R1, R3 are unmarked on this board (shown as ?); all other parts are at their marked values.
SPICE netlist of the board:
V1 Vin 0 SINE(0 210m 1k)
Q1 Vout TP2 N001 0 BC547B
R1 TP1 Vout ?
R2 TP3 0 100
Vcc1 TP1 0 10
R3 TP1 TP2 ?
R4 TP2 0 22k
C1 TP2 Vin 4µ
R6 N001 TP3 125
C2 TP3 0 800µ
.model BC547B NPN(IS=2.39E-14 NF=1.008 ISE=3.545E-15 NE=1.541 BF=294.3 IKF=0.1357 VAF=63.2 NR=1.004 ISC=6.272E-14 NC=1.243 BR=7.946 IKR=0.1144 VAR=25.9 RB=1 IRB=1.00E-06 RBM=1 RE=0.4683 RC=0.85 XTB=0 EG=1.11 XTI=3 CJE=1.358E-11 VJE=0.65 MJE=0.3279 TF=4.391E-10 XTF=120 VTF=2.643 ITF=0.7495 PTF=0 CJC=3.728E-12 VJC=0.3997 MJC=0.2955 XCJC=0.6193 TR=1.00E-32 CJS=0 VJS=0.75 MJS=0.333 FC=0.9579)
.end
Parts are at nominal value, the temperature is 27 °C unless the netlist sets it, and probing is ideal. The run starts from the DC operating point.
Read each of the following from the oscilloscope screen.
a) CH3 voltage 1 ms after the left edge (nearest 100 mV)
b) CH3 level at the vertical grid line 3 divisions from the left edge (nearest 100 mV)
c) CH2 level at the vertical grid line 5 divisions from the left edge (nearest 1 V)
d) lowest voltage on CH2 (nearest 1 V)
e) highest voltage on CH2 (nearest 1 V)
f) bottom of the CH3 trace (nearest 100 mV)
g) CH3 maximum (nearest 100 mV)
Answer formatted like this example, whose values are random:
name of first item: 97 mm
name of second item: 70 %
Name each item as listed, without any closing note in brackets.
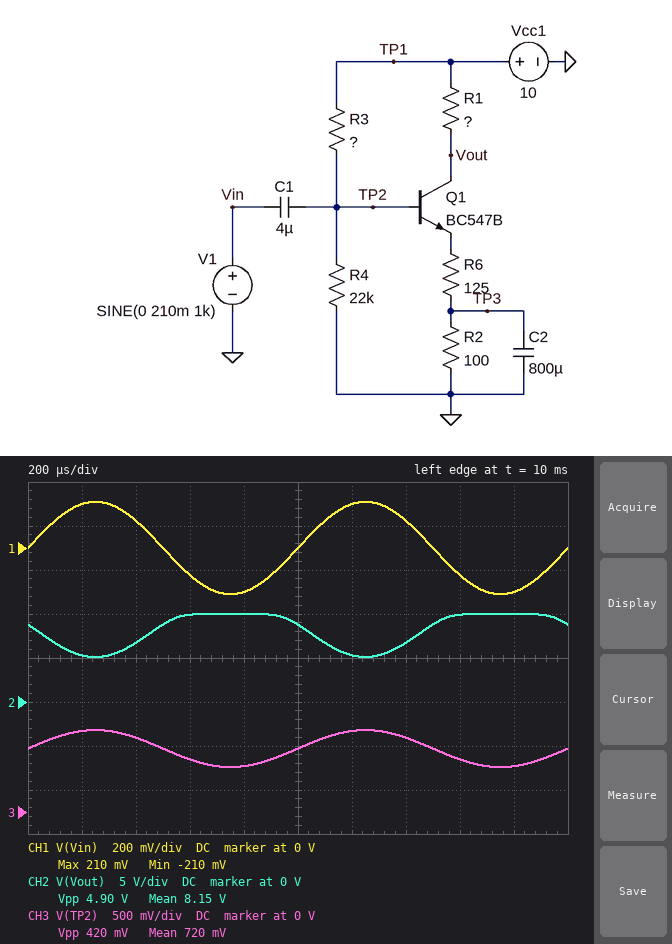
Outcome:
CH3 voltage 1 ms after the left edge: 700 mV
CH3 level at the vertical grid line 3 divisions from the left edge: 600 mV
CH2 level at the vertical grid line 5 divisions from the left edge: 9 V
lowest voltage on CH2: 5 V
highest voltage on CH2: 10 V
bottom of the CH3 trace: 500 mV
CH3 maximum: 900 mV
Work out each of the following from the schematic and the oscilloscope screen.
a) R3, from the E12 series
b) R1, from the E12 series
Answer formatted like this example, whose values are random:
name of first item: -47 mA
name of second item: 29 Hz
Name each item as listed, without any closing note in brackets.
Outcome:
R3, from the E12 series: 270 kΩ
R1, from the E12 series: 2.7 kΩ
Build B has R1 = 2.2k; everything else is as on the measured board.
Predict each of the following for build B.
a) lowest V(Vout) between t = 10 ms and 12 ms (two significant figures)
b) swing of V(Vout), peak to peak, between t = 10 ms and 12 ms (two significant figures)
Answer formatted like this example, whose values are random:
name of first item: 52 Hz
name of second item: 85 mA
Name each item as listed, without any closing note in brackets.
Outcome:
lowest V(Vout) between t = 10 ms and 12 ms: 6.0 V
swing of V(Vout), peak to peak, between t = 10 ms and 12 ms: 4.0 V
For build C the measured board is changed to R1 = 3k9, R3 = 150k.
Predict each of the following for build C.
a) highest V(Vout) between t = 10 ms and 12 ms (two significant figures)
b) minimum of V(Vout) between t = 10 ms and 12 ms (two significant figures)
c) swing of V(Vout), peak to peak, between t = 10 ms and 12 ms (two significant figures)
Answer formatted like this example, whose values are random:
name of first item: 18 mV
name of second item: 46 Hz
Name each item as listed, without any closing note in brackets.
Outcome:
highest V(Vout) between t = 10 ms and 12 ms: 9.7 V
minimum of V(Vout) between t = 10 ms and 12 ms: 570 mV
swing of V(Vout), peak to peak, between t = 10 ms and 12 ms: 9.1 V
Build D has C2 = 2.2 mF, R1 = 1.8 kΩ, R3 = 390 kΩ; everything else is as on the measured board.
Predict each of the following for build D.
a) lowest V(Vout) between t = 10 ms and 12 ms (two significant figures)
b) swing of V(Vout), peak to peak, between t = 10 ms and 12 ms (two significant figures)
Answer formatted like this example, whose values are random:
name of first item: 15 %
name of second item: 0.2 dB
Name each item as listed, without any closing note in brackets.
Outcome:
lowest V(Vout) between t = 10 ms and 12 ms: 8.5 V
swing of V(Vout), peak to peak, between t = 10 ms and 12 ms: 1.5 V
